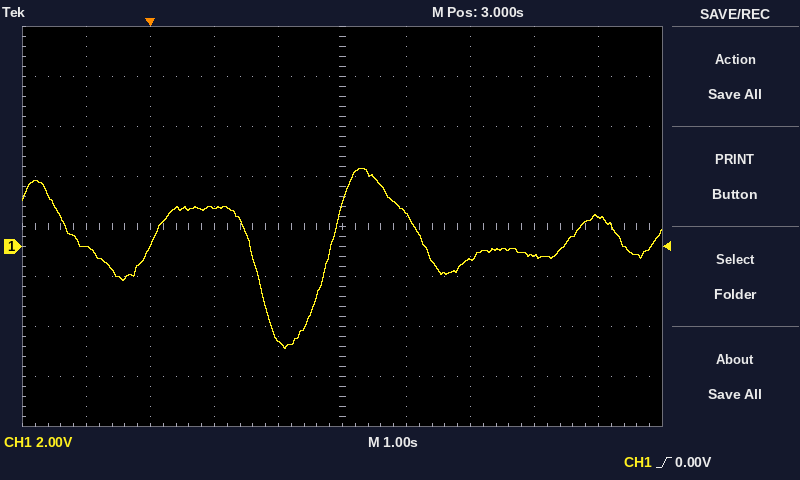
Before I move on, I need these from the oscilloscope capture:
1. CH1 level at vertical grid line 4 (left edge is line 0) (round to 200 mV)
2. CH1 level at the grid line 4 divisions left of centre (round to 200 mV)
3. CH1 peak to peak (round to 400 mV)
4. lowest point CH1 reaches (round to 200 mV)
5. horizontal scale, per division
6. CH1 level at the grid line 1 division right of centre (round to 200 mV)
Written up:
-3.8 V
0.0 V
7.2 V
-4.0 V
1 s
1.4 V
